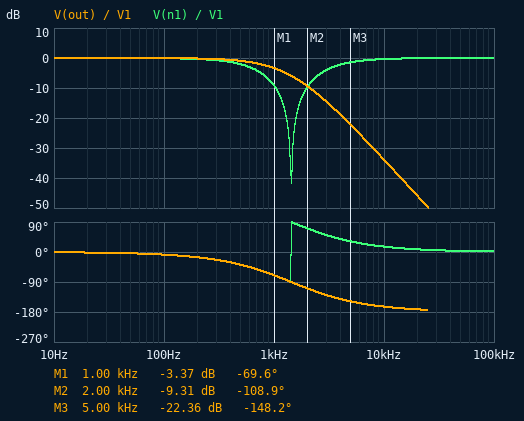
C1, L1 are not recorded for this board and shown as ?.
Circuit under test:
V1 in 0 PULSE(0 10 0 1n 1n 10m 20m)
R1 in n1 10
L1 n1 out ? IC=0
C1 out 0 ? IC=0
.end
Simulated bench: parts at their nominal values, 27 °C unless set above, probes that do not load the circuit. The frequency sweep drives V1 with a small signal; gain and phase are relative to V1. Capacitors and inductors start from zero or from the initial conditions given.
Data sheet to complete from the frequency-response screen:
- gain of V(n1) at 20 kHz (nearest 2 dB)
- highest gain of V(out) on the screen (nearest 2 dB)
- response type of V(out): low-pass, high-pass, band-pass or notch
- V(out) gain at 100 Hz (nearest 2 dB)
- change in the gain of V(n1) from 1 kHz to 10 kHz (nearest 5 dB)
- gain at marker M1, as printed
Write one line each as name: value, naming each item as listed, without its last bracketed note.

gain of V(n1) at 20 kHz: 0 dB
highest gain of V(out) on the screen: 0 dB
response type of V(out): low-pass, high-pass, band-pass or notch: low-pass
V(out) gain at 100 Hz: 0 dB
change in the gain of V(n1) from 1 kHz to 10 kHz: 10 dB
gain at marker M1, as printed: -3.37 dB
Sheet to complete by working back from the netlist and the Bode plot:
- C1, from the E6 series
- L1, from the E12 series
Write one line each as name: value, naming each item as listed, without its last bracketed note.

C1, from the E6 series: 22 µF
L1, from the E12 series: 560 µH
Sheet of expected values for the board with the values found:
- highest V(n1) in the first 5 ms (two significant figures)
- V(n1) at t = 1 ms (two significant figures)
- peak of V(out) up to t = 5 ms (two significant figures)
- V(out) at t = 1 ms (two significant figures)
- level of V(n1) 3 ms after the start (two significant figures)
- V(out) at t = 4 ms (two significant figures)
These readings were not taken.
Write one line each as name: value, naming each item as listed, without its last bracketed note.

highest V(n1) in the first 5 ms: 10 V
V(n1) at t = 1 ms: 10 V
peak of V(out) up to t = 5 ms: 10 V
V(out) at t = 1 ms: 10 V
level of V(n1) 3 ms after the start: 10 V
V(out) at t = 4 ms: 10 V
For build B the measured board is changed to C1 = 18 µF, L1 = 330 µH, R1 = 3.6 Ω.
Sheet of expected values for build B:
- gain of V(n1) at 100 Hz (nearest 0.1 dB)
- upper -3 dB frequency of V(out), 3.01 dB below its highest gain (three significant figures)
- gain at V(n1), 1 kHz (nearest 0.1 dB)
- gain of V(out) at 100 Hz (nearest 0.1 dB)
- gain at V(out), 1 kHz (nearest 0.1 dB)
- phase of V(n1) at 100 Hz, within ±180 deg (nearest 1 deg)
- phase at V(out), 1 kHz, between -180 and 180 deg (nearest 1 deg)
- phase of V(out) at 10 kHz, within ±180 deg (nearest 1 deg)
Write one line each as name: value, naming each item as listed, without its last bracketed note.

gain of V(n1) at 100 Hz: 0 dB
upper -3 dB frequency of V(out), 3.01 dB below its highest gain: 2.45 kHz
gain at V(n1), 1 kHz: -1.1 dB
gain of V(out) at 100 Hz: 0 dB
gain at V(out), 1 kHz: 1.2 dB
phase of V(n1) at 100 Hz, within ±180 deg: -2 deg
phase at V(out), 1 kHz, between -180 and 180 deg: -28 deg
phase of V(out) at 10 kHz, within ±180 deg: -170 deg
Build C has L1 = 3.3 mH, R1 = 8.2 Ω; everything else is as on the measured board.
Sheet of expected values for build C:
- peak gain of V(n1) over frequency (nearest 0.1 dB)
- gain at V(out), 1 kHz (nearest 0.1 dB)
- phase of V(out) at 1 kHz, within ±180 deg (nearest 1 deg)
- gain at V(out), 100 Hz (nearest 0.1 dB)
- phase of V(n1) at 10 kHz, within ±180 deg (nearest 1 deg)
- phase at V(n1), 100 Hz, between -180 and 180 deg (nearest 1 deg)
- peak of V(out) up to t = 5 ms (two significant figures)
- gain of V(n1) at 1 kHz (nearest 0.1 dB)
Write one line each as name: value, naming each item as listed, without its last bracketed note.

peak gain of V(n1) over frequency: 0 dB
gain at V(out), 1 kHz: -6.8 dB
phase of V(out) at 1 kHz, within ±180 deg: -149 deg
gain at V(out), 100 Hz: 0.2 dB
phase of V(n1) at 10 kHz, within ±180 deg: 2 deg
phase at V(n1), 100 Hz, between -180 and 180 deg: -7 deg
peak of V(out) up to t = 5 ms: 13 V
gain of V(n1) at 1 kHz: -1.4 dB
